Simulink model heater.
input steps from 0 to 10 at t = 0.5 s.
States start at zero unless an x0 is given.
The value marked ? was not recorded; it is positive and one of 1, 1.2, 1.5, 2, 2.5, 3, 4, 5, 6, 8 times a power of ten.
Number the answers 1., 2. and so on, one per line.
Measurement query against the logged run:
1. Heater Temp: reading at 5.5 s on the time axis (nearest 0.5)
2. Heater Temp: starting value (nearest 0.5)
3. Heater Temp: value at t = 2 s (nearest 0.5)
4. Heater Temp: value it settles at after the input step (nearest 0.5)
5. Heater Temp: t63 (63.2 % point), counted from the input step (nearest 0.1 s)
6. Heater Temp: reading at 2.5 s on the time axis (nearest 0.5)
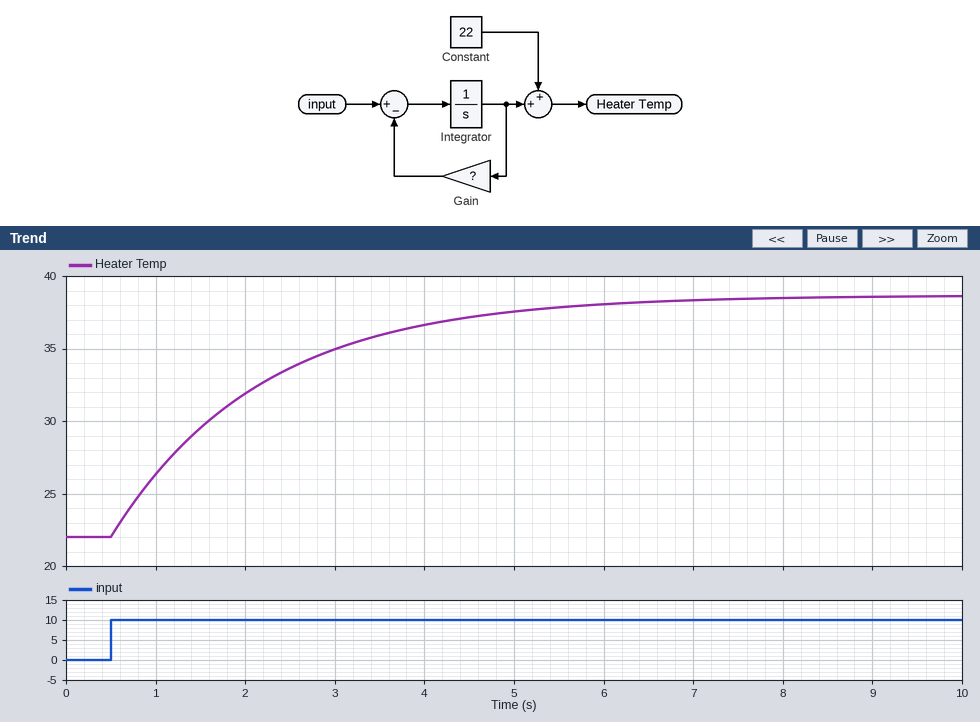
1. 38.0
2. 22.0
3. 32.0
4. 38.5
5. 1.7 s
6. 33.5
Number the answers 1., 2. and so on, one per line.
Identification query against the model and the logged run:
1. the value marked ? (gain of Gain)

1. 0.6
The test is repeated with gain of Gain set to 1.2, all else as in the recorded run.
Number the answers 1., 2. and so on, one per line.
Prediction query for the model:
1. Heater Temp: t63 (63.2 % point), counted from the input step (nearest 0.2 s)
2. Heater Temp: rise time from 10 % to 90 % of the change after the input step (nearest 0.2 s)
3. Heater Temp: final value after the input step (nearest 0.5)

1. 0.8 s
2. 1.8 s
3. 30.5
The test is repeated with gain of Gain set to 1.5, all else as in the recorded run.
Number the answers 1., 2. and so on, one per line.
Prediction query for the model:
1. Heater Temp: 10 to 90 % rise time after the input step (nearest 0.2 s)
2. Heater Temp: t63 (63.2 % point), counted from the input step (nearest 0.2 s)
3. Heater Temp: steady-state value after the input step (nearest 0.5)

1. 1.4 s
2. 0.6 s
3. 28.5
